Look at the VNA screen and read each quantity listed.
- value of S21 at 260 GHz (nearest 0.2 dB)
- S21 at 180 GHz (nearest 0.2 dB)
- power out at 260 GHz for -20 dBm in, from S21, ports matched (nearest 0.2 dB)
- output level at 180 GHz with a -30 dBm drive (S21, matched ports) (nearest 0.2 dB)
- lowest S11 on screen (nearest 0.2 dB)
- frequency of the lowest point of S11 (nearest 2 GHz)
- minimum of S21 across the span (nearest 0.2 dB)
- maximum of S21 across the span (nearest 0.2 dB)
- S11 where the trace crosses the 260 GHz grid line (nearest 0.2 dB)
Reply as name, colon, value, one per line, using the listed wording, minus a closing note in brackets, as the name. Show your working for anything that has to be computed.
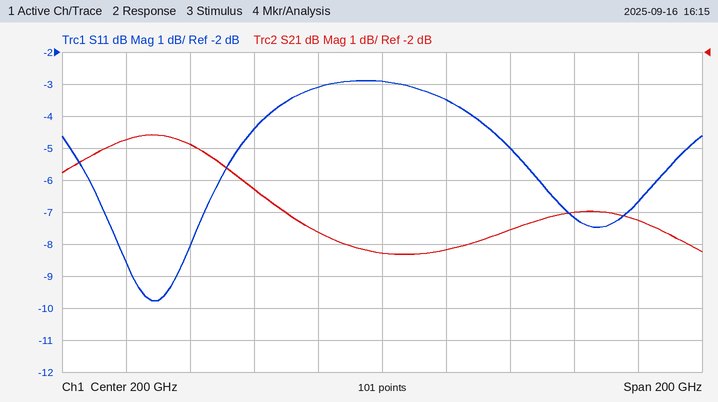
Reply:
value of S21 at 260 GHz: -7.0 dB
S21 at 180 GHz: -7.6 dB
power out at 260 GHz for -20 dBm in, from S21, ports matched: -20 dBm + (-7.0 dB) = -27.0 dBm
output level at 180 GHz with a -30 dBm drive (S21, matched ports): -30 dBm + (-7.6 dB) = -37.6 dBm
lowest S11 on screen: -9.8 dB
frequency of the lowest point of S11: 128 GHz
minimum of S21 across the span: -8.4 dB
maximum of S21 across the span: -4.6 dB
S11 where the trace crosses the 260 GHz grid line: -7.2 dB
